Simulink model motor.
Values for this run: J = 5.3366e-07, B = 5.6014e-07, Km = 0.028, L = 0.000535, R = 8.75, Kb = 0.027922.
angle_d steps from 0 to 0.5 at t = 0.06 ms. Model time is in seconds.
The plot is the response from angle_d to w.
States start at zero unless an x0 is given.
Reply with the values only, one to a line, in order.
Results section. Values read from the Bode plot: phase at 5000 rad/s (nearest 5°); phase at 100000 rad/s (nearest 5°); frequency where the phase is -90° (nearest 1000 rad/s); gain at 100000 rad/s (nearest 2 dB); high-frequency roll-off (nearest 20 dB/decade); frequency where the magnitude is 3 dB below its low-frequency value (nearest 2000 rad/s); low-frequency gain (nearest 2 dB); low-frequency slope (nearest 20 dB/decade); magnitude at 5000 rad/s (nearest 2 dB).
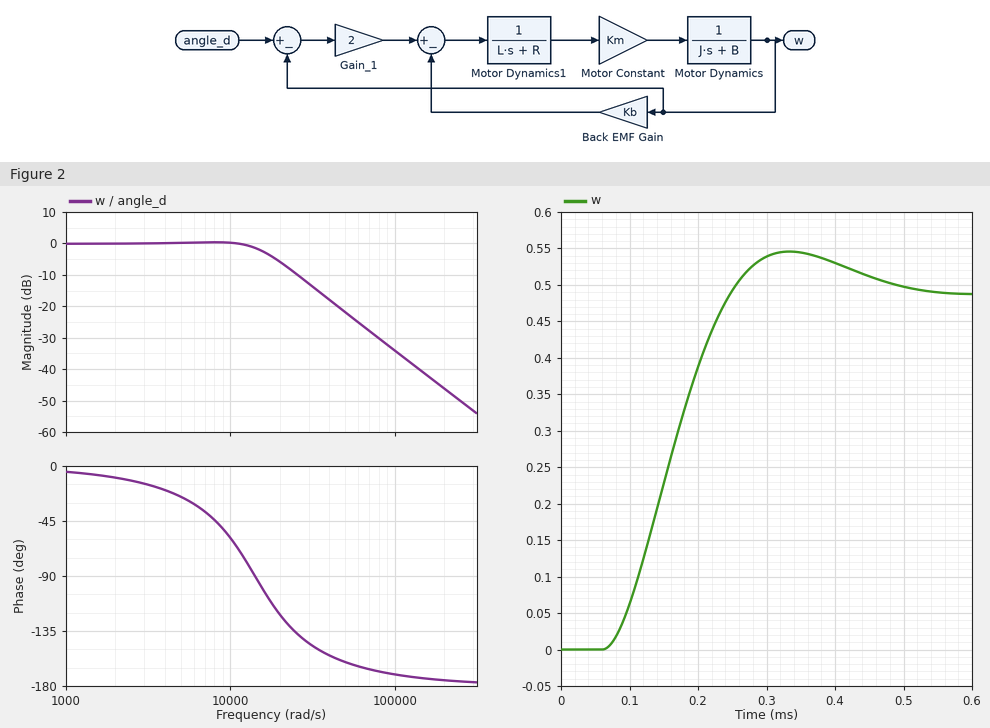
-25°
-170°
14000 rad/s
-34 dB
-40 dB/decade
16000 rad/s
0 dB
0 dB/decade
0 dB
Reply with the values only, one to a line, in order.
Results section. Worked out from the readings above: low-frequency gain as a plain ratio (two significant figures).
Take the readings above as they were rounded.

1.0
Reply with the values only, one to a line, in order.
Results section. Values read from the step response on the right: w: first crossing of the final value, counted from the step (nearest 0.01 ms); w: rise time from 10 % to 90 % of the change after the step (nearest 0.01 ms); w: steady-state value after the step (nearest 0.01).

0.19 ms
0.13 ms
0.49
